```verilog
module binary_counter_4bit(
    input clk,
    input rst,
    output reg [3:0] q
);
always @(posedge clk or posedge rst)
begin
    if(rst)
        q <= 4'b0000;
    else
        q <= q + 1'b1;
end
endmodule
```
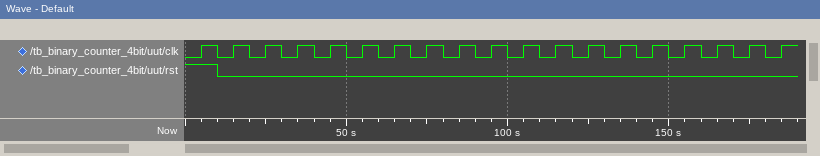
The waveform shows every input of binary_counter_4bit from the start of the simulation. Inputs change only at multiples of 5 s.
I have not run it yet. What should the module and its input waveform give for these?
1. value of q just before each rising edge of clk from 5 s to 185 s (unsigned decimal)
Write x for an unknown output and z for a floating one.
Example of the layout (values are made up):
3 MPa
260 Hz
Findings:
0, 0, 1, 2, 3, 4, 5, 6, 7, 8, 9, 10, 11, 12, 13, 14, 15, 0, 1
